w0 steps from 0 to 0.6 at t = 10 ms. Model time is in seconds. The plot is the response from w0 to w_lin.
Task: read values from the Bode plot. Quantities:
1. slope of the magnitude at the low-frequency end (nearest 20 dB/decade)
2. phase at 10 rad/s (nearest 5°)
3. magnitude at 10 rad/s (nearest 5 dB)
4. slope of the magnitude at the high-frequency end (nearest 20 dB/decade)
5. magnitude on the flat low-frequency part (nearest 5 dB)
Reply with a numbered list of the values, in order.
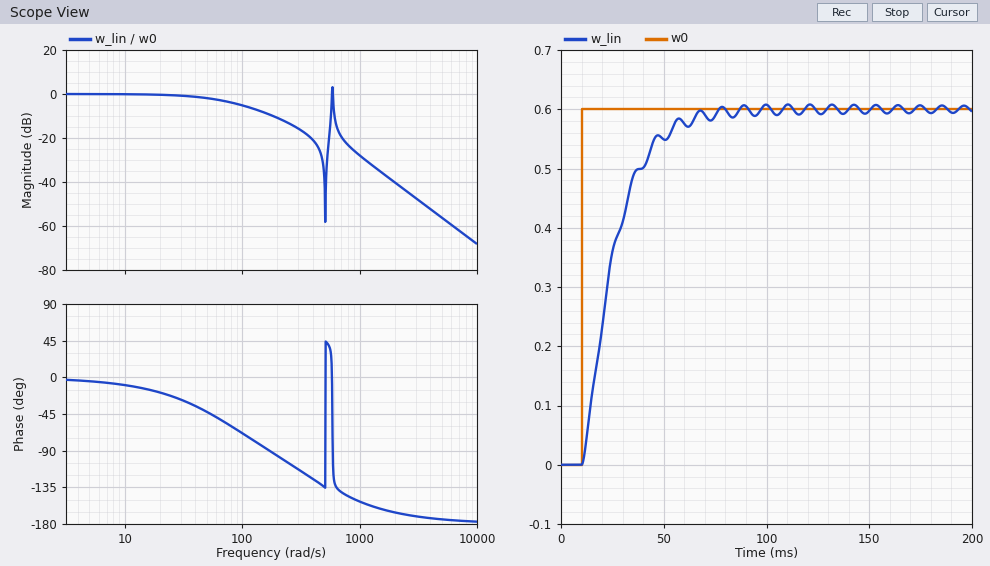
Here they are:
1. 0 dB/decade
2. -10°
3. 0 dB
4. -40 dB/decade
5. 0 dB
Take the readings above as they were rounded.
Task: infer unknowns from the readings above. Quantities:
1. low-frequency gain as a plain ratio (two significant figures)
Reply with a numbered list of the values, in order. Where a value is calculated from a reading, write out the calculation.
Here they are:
1. 10^(0 / 20) = 1.0
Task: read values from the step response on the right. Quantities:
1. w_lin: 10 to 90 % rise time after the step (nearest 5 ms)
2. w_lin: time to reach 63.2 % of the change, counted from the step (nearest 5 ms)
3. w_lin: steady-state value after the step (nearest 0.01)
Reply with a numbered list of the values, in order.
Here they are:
1. 30 ms
2. 15 ms
3. 0.60
